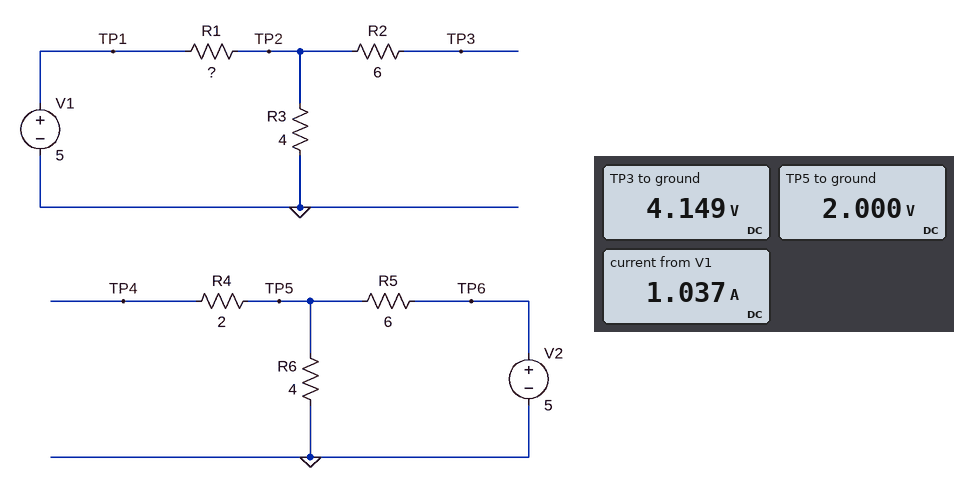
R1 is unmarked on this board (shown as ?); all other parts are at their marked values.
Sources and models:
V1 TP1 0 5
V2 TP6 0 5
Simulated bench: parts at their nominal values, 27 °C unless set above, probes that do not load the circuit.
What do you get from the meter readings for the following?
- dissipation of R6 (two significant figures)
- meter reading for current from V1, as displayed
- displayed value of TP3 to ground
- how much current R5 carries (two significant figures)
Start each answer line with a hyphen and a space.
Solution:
- 1.0 W
- 1.037 A
- 4.149 V
- 500 mA
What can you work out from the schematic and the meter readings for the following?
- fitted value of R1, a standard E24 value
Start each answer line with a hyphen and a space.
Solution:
- 0.82 Ω
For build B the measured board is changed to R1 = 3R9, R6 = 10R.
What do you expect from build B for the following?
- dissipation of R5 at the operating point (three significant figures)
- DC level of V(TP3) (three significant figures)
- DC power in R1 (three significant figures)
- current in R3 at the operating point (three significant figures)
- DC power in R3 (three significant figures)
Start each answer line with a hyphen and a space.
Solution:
- 586 mW
- 2.53 V
- 1.56 W
- 633 mA
- 1.60 W
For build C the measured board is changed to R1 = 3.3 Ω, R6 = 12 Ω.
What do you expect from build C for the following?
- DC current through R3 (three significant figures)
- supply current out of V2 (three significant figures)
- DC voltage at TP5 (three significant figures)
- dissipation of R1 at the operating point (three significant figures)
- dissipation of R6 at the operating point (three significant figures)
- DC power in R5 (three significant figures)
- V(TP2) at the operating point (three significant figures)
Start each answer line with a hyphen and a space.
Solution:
- 685 mA
- 278 mA
- 3.33 V
- 1.55 W
- 926 mW
- 463 mW
- 2.74 V
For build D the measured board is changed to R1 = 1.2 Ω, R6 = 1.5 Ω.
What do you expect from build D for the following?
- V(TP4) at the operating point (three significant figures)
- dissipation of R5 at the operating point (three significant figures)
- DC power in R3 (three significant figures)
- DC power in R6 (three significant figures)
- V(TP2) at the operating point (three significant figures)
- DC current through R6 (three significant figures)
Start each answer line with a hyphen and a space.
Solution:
- 1.00 V
- 2.67 W
- 3.70 W
- 667 mW
- 3.85 V
- 667 mA
